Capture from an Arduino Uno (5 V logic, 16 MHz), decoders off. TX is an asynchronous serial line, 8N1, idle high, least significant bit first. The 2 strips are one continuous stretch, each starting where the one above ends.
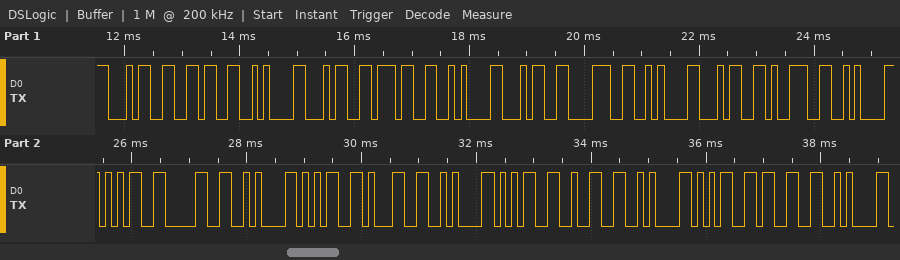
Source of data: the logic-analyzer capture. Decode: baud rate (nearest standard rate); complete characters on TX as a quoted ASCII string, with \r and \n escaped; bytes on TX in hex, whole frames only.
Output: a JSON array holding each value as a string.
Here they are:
["9600 baud", "\"46\\n47\\n48\\n49\\n50\\n51\\n52\\n53\\n\"", "34 36 0A 34 37 0A 34 38 0A 34 39 0A 35 30 0A 35 31 0A 35 32 0A 35 33 0A"]
